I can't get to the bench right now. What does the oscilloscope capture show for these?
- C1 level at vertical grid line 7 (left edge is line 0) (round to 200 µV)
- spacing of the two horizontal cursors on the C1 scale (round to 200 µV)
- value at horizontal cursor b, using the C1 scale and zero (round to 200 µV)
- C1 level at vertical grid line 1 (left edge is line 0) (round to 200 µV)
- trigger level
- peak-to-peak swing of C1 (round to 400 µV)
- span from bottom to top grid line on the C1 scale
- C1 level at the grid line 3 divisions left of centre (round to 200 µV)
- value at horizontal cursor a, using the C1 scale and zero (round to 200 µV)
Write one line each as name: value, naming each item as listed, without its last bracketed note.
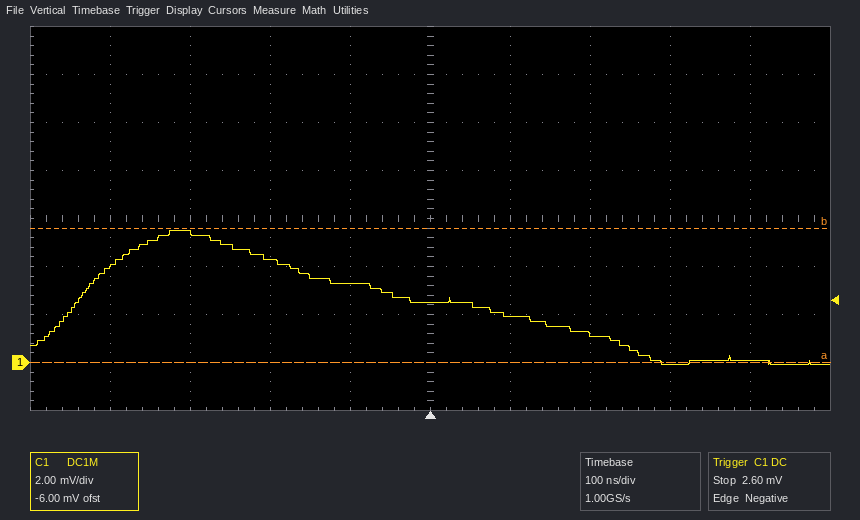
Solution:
C1 level at vertical grid line 7 (left edge is line 0): 1.2 mV
spacing of the two horizontal cursors on the C1 scale: 5.6 mV
value at horizontal cursor b, using the C1 scale and zero: 5.6 mV
C1 level at vertical grid line 1 (left edge is line 0): 4.0 mV
trigger level: 2.60 mV
peak-to-peak swing of C1: 5.6 mV
span from bottom to top grid line on the C1 scale: 16 mV
C1 level at the grid line 3 divisions left of centre: 5.4 mV
value at horizontal cursor a, using the C1 scale and zero: 0.0 mV
